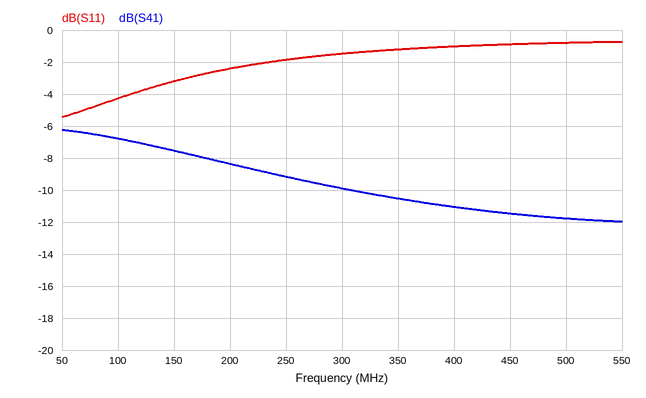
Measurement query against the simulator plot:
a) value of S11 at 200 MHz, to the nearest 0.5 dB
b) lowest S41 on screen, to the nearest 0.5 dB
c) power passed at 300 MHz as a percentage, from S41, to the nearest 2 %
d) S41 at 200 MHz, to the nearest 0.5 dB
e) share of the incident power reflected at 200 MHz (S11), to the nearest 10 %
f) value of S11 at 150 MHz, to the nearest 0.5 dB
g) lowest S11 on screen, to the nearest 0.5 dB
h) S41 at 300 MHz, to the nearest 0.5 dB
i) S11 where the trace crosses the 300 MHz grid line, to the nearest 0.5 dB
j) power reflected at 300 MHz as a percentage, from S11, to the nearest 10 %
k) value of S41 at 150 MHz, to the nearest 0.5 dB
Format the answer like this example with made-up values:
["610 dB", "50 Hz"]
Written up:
["-2.5 dB", "-12.0 dB", "10 %", "-8.5 dB", "60 %", "-3.0 dB", "-5.5 dB", "-10.0 dB", "-1.5 dB", "70 %", "-7.5 dB"]
